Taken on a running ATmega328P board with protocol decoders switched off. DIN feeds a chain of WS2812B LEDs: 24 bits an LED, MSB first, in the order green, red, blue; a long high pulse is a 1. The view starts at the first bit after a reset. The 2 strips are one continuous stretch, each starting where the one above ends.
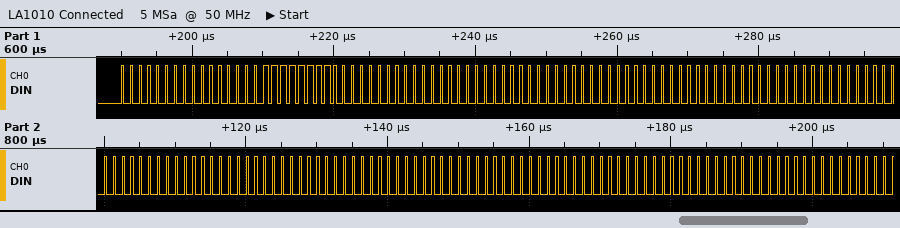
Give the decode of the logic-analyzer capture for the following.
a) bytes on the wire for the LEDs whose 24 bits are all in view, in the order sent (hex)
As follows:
00 00 FF 00 00 00 00 00 00 00 00 00 00 00 00 00 00 00 00 00 00
